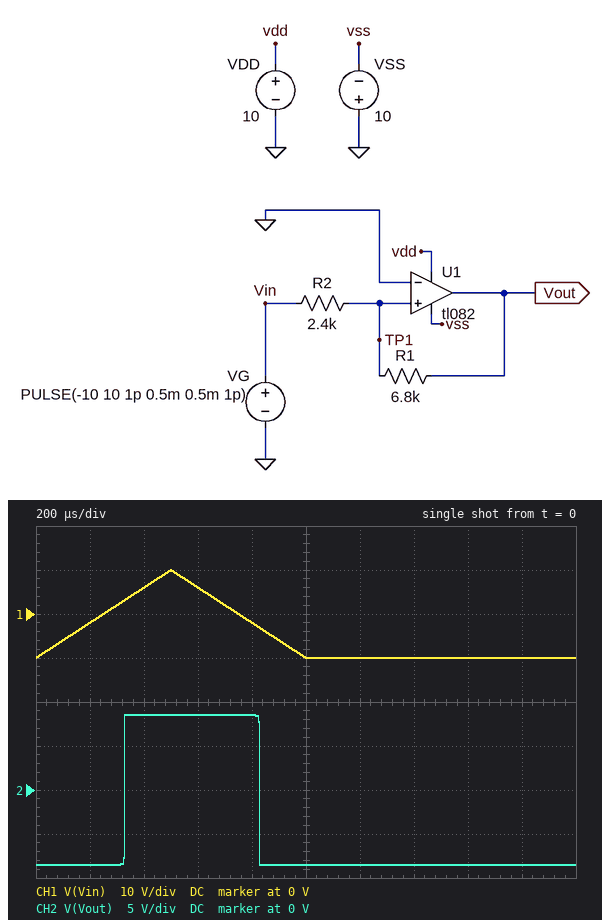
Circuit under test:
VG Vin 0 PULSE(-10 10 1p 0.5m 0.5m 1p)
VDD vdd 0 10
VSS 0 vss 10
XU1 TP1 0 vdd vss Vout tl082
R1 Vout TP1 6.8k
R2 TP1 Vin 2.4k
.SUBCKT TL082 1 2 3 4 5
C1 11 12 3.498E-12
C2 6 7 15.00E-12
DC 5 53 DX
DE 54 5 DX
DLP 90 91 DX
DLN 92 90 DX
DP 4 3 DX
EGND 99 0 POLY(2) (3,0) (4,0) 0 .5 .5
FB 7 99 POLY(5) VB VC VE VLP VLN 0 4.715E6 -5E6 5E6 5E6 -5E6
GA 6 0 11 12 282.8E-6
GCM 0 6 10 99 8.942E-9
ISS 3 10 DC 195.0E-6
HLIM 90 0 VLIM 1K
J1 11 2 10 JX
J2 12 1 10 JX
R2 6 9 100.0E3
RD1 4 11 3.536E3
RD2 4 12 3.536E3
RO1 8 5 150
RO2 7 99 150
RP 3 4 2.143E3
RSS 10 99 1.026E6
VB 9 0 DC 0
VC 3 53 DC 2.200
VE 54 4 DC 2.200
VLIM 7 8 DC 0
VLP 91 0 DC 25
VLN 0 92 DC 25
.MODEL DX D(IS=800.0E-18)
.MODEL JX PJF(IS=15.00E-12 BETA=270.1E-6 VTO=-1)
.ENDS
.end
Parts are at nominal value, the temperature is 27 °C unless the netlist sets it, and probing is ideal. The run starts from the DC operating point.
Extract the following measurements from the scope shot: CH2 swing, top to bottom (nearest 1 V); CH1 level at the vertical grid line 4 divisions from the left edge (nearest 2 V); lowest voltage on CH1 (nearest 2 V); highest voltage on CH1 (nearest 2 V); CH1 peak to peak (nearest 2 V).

17 V
-2 V
-10 V
10 V
20 V
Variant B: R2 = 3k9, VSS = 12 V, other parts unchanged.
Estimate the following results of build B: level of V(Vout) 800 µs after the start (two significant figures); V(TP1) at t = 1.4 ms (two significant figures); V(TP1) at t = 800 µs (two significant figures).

8.5 V
-10 V
1.8 V
